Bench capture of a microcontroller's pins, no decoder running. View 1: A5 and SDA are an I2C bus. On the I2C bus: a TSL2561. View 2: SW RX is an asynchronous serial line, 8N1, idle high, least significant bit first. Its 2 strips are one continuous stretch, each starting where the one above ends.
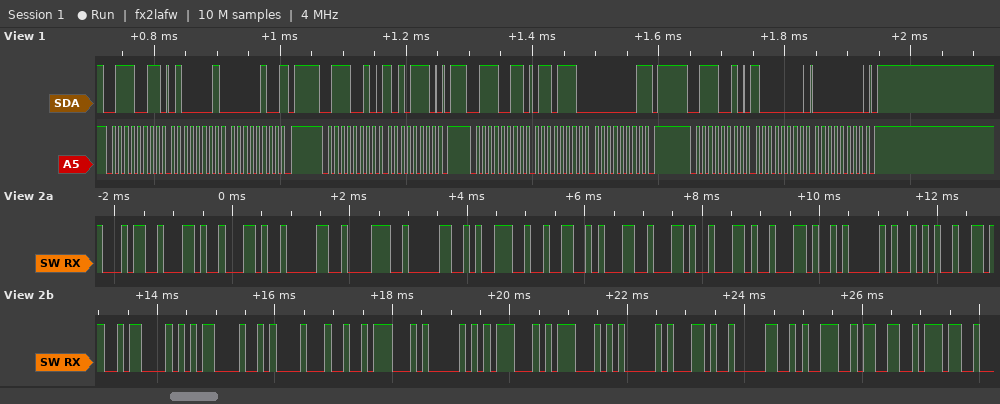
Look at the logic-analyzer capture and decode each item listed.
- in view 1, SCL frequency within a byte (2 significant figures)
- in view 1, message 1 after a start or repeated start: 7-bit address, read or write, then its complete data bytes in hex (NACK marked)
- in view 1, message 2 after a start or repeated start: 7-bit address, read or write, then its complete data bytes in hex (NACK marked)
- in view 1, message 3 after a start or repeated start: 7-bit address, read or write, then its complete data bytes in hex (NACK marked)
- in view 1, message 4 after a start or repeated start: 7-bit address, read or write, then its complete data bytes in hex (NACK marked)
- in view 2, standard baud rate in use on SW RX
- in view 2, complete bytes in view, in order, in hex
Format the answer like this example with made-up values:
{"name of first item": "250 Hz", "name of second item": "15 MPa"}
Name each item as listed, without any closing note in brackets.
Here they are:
{"in view 1, SCL frequency within a byte": "100 kHz", "in view 1, message 1 after a start or repeated start: 7-bit address, read or write, then its complete data bytes in hex": "0x39 read: 41 04 NACK", "in view 1, message 2 after a start or repeated start: 7-bit address, read or write, then its complete data bytes in hex": "0x39 write: AE", "in view 1, message 3 after a start or repeated start: 7-bit address, read or write, then its complete data bytes in hex": "0x39 read: 6E 01 NACK", "in view 1, message 4 after a start or repeated start: 7-bit address, read or write, then its complete data bytes in hex": "0x39 write: 80 00", "in view 2, standard baud rate in use on SW RX": "9600 baud", "in view 2, complete bytes in view, in order, in hex": "34 2C 2C 30 38 30 39 32 31 2C 2C 2C 41 2A 36 43 0D 0A 24 47 50 47 47 41 2C 30 39 33 37"}
